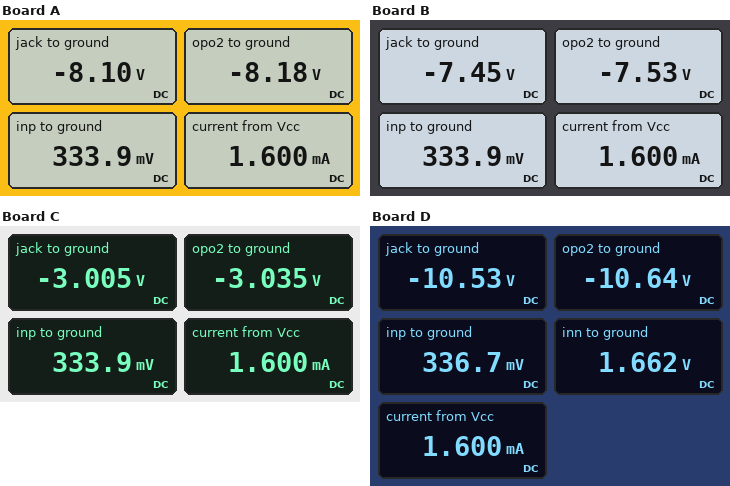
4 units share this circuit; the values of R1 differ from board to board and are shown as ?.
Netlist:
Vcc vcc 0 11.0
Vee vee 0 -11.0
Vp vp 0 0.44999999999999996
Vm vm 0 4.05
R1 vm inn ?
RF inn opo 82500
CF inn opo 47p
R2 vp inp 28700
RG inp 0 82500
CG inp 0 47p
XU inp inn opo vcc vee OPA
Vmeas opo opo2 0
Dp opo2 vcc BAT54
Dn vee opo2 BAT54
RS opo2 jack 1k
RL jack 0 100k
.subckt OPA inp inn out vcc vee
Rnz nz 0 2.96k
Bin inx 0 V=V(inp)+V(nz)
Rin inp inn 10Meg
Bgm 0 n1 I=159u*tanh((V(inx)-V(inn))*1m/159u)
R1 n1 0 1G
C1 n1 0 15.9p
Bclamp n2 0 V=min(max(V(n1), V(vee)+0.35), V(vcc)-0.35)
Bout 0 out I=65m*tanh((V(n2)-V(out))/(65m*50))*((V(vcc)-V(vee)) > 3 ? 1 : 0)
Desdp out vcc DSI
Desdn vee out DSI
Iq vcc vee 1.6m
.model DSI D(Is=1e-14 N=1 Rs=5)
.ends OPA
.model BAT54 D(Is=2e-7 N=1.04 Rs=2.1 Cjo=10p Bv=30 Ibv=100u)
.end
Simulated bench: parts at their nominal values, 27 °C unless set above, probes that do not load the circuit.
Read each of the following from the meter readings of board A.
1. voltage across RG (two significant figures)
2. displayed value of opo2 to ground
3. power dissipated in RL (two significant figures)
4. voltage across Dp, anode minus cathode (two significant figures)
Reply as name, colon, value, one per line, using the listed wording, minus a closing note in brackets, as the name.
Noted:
voltage across RG: 330 mV
displayed value of opo2 to ground: -8.18 V
power dissipated in RL: 660 µW
voltage across Dp, anode minus cathode: -19 V
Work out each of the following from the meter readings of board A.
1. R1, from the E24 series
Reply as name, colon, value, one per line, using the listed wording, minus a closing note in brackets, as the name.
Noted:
R1, from the E24 series: 36 kΩ
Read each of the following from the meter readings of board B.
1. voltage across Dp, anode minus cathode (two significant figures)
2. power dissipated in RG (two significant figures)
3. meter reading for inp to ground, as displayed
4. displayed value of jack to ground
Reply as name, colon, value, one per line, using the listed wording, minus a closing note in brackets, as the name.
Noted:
voltage across Dp, anode minus cathode: -19 V
power dissipated in RG: 1.4 µW
meter reading for inp to ground, as displayed: 333.9 mV
displayed value of jack to ground: -7.45 V
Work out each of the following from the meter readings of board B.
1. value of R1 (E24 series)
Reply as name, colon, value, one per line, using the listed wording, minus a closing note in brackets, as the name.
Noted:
value of R1: 39 kΩ
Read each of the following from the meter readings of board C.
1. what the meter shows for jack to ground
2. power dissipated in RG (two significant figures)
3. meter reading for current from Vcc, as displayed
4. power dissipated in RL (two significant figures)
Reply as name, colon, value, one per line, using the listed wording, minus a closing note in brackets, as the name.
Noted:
what the meter shows for jack to ground: -3.005 V
power dissipated in RG: 1.4 µW
meter reading for current from Vcc, as displayed: 1.600 mA
power dissipated in RL: 90 µW
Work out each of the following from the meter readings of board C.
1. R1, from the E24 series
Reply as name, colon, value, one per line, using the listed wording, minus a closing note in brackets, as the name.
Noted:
R1, from the E24 series: 91 kΩ
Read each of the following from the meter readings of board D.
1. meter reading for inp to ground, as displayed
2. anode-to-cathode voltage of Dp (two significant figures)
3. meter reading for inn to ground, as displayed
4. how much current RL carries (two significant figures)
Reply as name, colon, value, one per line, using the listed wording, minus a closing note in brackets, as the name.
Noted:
meter reading for inp to ground, as displayed: 336.7 mV
anode-to-cathode voltage of Dp: -22 V
meter reading for inn to ground, as displayed: 1.662 V
how much current RL carries: 110 µA
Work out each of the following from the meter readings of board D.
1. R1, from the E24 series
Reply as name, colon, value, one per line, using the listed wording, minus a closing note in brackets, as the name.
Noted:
R1, from the E24 series: 16 kΩ
